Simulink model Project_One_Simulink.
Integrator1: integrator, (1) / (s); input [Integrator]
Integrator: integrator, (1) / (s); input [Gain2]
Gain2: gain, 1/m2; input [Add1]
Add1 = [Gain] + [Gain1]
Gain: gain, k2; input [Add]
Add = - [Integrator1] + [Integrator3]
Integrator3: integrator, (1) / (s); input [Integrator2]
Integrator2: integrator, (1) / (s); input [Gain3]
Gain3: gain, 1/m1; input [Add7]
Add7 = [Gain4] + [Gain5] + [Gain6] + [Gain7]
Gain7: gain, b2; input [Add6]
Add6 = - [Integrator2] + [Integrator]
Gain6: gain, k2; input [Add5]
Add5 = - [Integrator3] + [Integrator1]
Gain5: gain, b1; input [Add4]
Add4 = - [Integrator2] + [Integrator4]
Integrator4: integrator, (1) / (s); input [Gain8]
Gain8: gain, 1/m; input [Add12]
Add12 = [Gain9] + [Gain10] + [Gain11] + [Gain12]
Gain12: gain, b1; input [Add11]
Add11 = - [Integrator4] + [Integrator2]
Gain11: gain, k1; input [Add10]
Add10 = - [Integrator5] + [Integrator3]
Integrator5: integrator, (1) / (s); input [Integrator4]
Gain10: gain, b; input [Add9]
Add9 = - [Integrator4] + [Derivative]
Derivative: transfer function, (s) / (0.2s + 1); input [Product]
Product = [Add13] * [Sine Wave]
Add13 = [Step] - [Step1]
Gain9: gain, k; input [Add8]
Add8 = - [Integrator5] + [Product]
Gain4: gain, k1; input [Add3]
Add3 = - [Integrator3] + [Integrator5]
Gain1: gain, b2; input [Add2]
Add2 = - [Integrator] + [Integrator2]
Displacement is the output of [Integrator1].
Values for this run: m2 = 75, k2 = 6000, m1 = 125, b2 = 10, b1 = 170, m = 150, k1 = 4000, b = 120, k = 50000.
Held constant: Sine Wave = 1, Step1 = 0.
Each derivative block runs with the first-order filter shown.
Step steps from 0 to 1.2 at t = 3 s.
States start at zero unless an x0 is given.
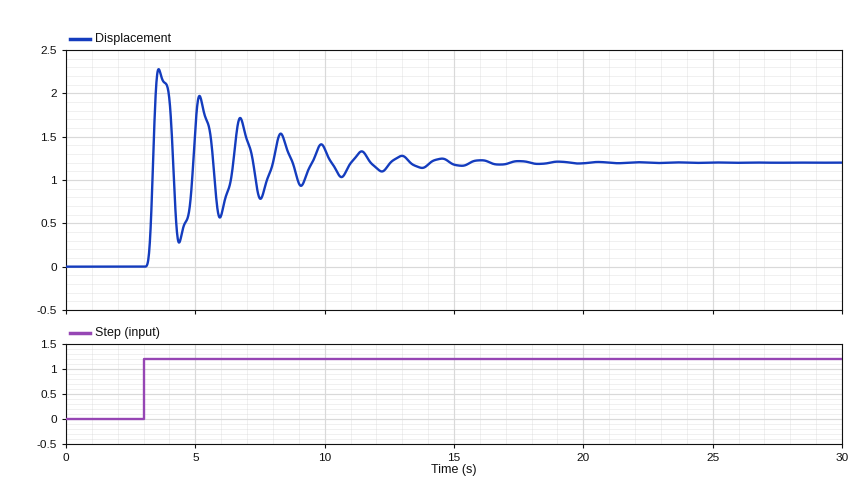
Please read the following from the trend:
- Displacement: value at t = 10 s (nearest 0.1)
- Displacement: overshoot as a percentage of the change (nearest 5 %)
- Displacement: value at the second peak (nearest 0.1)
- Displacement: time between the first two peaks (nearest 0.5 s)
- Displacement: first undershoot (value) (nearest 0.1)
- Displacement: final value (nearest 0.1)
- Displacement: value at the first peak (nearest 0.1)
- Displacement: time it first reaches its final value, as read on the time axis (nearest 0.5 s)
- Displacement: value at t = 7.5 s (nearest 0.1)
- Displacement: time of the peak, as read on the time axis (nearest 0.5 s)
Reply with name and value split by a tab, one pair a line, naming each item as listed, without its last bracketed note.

Displacement: value at t = 10 s	1.4
Displacement: overshoot as a percentage of the change	90 %
Displacement: value at the second peak	2.0
Displacement: time between the first two peaks	1.5 s
Displacement: first undershoot (value)	0.3
Displacement: final value	1.2
Displacement: value at the first peak	2.3
Displacement: time it first reaches its final value, as read on the time axis	3.5 s
Displacement: value at t = 7.5 s	0.8
Displacement: time of the peak, as read on the time axis	3.5 s
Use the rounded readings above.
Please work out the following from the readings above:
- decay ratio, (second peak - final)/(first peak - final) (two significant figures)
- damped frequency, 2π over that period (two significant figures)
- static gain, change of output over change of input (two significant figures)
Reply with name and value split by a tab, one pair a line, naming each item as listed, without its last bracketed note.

decay ratio, (second peak - final)/(first peak - final)	0.73
damped frequency, 2π over that period	4.2 rad/s
static gain, change of output over change of input	1.0
